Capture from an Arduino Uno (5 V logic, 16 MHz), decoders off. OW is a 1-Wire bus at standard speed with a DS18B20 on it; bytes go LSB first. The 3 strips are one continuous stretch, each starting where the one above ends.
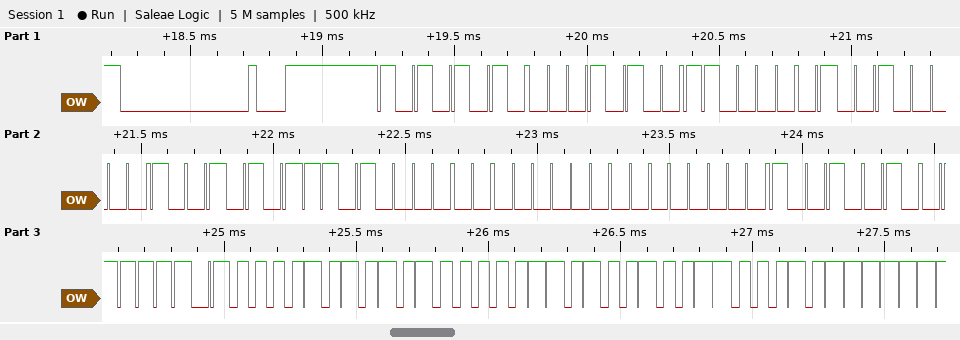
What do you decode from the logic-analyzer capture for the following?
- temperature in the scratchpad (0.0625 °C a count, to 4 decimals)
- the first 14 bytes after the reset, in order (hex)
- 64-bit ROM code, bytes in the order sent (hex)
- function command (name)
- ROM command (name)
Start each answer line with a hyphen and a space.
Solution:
- 85.0000 °C
- 55 28 83 04 A9 0B 00 00 49 BE 50 05 4B 46
- 28 83 04 A9 0B 00 00 49
- Read Scratchpad
- Match ROM
